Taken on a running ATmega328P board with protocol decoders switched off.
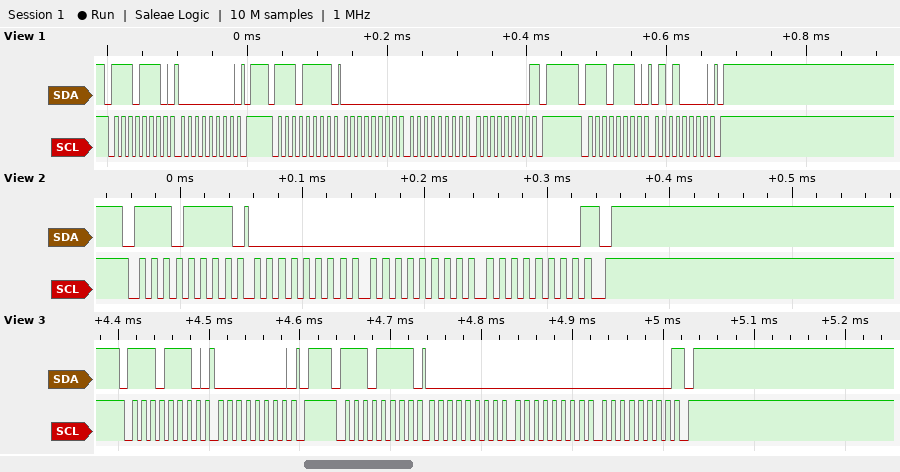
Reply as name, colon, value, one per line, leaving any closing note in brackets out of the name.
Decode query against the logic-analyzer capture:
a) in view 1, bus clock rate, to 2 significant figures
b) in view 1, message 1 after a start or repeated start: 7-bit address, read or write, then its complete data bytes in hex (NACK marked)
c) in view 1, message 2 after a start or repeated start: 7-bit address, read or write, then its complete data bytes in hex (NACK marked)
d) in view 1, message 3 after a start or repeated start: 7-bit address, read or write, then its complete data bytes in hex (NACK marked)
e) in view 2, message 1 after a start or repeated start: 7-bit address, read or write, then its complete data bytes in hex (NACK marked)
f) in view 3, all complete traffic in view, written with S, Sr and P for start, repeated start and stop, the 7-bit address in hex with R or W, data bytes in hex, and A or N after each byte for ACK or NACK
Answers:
in view 1, bus clock rate, to 2 significant figures: 100 kHz
in view 1, message 1 after a start or repeated start: 7-bit address, read or write, then its complete data bytes in hex: 0x77 write: 00
in view 1, message 2 after a start or repeated start: 7-bit address, read or write, then its complete data bytes in hex: 0x77 read: 00 00 00 NACK
in view 1, message 3 after a start or repeated start: 7-bit address, read or write, then its complete data bytes in hex: 0x77 write: 50
in view 2, message 1 after a start or repeated start: 7-bit address, read or write, then its complete data bytes in hex: 0x77 read: 00 00 00 NACK
in view 3, all complete traffic in view, written with S, Sr and P for start, repeated start and stop, the 7-bit address in hex with R or W, data bytes in hex, and A or N after each byte for ACK or NACK: S 77W A 00 A P S 77R A 00 A 00 A 00 N P
